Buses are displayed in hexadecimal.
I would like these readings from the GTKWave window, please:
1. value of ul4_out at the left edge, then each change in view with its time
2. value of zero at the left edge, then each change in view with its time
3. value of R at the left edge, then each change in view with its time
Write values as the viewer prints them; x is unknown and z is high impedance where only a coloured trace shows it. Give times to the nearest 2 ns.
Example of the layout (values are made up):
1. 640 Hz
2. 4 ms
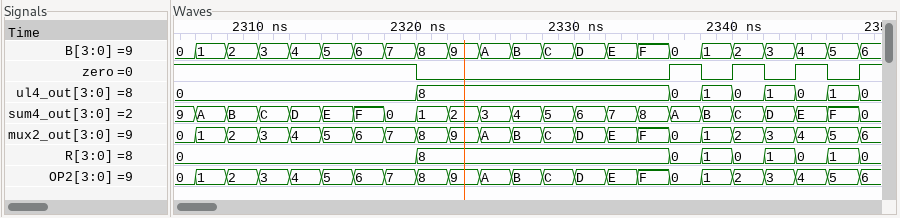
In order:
1. 0, 8 at 2320 ns, 0 at 2336 ns, 1 at 2338 ns, 0 at 2340 ns, 1 at 2342 ns, 0 at 2344 ns, 1 at 2346 ns, 0 at 2348 ns
2. 1, 0 at 2320 ns, 1 at 2336 ns, 0 at 2338 ns, 1 at 2340 ns, 0 at 2342 ns, 1 at 2344 ns, 0 at 2346 ns, 1 at 2348 ns
3. 0, 8 at 2320 ns, 0 at 2336 ns, 1 at 2338 ns, 0 at 2340 ns, 1 at 2342 ns, 0 at 2344 ns, 1 at 2346 ns, 0 at 2348 ns
